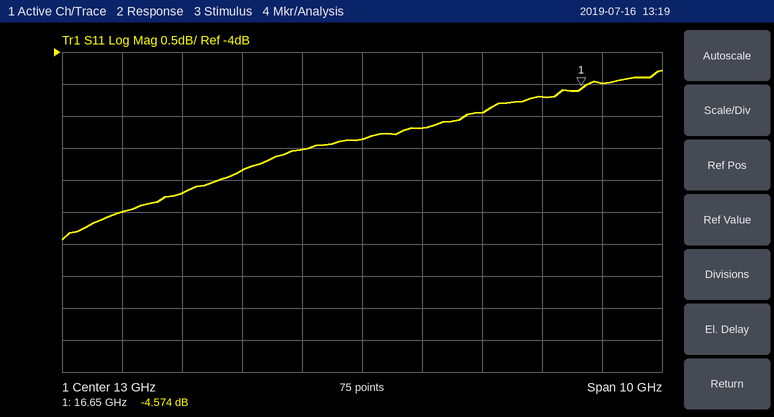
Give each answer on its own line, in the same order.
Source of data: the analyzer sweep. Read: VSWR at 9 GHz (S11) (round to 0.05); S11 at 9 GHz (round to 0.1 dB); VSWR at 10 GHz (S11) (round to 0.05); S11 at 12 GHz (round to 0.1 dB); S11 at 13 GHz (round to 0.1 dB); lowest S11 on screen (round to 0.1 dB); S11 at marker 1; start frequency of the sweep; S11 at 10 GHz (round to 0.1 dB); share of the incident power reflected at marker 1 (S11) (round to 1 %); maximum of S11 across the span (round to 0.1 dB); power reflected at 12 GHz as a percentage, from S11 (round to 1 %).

2.80
-6.5 dB
2.90
-5.5 dB
-5.4 dB
-6.9 dB
-4.574 dB
8 GHz
-6.2 dB
35 %
-4.3 dB
28 %
